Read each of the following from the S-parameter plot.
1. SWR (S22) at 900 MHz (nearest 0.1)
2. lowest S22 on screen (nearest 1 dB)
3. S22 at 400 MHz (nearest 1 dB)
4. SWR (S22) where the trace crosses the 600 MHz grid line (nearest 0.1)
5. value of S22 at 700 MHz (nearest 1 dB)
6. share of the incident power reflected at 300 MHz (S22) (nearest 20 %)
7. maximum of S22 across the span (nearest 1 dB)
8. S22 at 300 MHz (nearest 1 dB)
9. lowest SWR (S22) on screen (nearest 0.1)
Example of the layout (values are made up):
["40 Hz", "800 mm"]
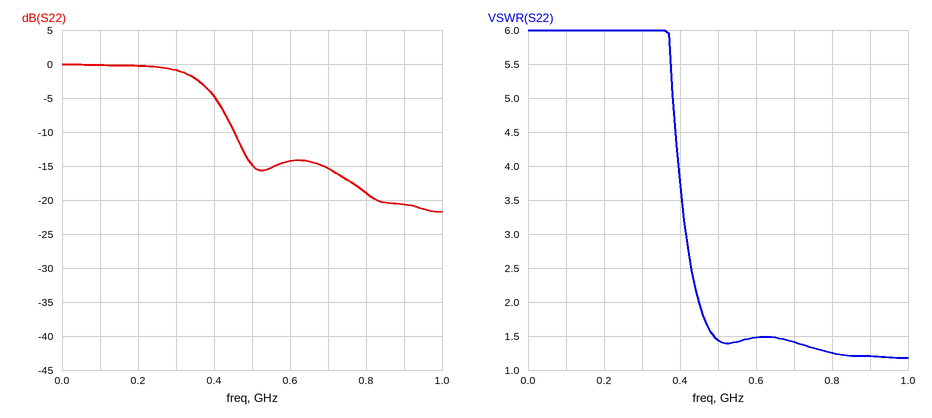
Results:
["1.2", "-22 dB", "-5 dB", "1.5", "-15 dB", "80 %", "0 dB", "-1 dB", "1.2"]
